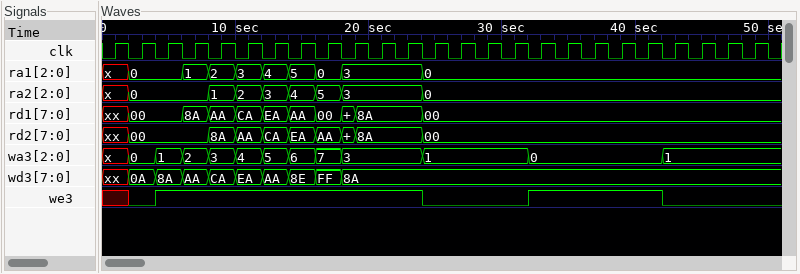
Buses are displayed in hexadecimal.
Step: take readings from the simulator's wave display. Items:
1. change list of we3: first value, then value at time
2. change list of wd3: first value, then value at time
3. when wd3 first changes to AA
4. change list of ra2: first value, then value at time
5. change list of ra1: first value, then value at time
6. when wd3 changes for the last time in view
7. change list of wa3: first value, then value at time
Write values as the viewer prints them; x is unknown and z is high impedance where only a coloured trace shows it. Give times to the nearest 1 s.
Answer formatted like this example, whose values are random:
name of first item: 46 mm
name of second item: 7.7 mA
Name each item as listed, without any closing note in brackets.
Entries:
change list of we3: first value, then value at time: x, 0 at 2 s, 1 at 4 s, 0 at 24 s, 1 at 32 s, 0 at 42 s
change list of wd3: first value, then value at time: xx, 0A at 2 s, 8A at 4 s, AA at 6 s, CA at 8 s, EA at 10 s, AA at 12 s, 8E at 14 s, FF at 16 s, 8A at 18 s
when wd3 first changes to AA: 6 s
change list of ra2: first value, then value at time: x, 0 at 2 s, 1 at 8 s, 2 at 10 s, 3 at 12 s, 4 at 14 s, 5 at 16 s, 3 at 18 s, 0 at 24 s
change list of ra1: first value, then value at time: x, 0 at 2 s, 1 at 6 s, 2 at 8 s, 3 at 10 s, 4 at 12 s, 5 at 14 s, 0 at 16 s, 3 at 18 s, 0 at 24 s
when wd3 changes for the last time in view: 18 s
change list of wa3: first value, then value at time: x, 0 at 2 s, 1 at 4 s, 2 at 6 s, 3 at 8 s, 4 at 10 s, 5 at 12 s, 6 at 14 s, 7 at 16 s, 3 at 18 s, 1 at 24 s, 0 at 32 s, 1 at 42 s
